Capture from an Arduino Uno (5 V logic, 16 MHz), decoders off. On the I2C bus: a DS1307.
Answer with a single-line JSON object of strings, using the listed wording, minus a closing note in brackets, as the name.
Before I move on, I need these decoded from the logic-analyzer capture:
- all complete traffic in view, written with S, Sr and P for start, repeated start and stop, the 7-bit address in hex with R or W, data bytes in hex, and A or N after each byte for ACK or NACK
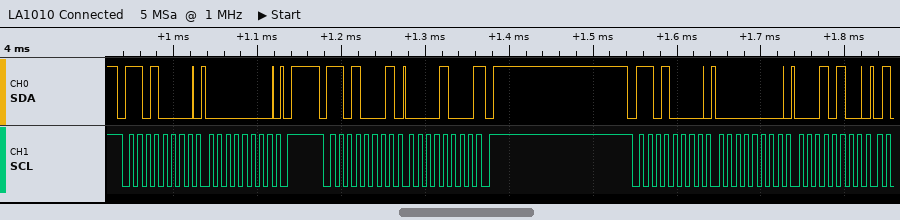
{"all complete traffic in view, written with S, Sr and P for start, repeated start and stop, the 7-bit address in hex with R or W, data bytes in hex, and A or N after each byte for ACK or NACK": "S 68W A 00 A P S 68R A 08 N P S 68W A 00 A 14 A"}
